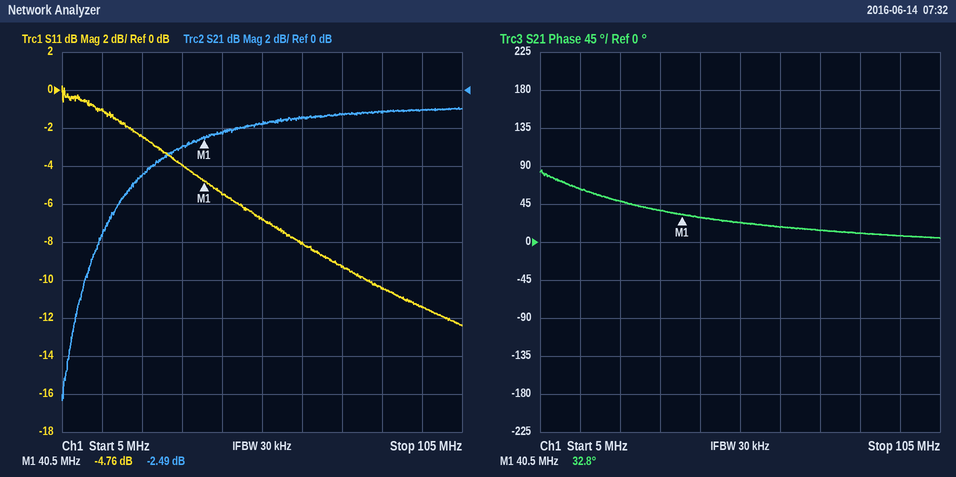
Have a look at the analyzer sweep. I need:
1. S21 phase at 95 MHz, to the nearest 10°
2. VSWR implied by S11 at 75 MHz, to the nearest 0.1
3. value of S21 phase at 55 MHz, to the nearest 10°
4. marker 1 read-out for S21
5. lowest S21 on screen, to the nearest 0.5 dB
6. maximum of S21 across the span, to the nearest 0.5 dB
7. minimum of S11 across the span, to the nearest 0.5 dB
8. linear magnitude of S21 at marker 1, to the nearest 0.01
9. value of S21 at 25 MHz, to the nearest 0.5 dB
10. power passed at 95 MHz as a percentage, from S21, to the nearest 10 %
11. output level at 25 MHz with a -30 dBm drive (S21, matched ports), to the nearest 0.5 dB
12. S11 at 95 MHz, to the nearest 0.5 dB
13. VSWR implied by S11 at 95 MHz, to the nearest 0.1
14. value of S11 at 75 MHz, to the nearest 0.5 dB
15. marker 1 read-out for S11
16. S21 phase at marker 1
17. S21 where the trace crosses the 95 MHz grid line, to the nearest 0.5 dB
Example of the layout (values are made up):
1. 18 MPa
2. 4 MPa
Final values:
1. 10°
2. 2.0
3. 20°
4. -2.49 dB
5. -16.5 dB
6. -1.0 dB
7. -12.5 dB
8. 0.75
9. -4.5 dB
10. 80 %
11. -34.5 dBm
12. -11.5 dB
13. 1.7
14. -9.5 dB
15. -4.76 dB
16. 32.8°
17. -1.0 dB
